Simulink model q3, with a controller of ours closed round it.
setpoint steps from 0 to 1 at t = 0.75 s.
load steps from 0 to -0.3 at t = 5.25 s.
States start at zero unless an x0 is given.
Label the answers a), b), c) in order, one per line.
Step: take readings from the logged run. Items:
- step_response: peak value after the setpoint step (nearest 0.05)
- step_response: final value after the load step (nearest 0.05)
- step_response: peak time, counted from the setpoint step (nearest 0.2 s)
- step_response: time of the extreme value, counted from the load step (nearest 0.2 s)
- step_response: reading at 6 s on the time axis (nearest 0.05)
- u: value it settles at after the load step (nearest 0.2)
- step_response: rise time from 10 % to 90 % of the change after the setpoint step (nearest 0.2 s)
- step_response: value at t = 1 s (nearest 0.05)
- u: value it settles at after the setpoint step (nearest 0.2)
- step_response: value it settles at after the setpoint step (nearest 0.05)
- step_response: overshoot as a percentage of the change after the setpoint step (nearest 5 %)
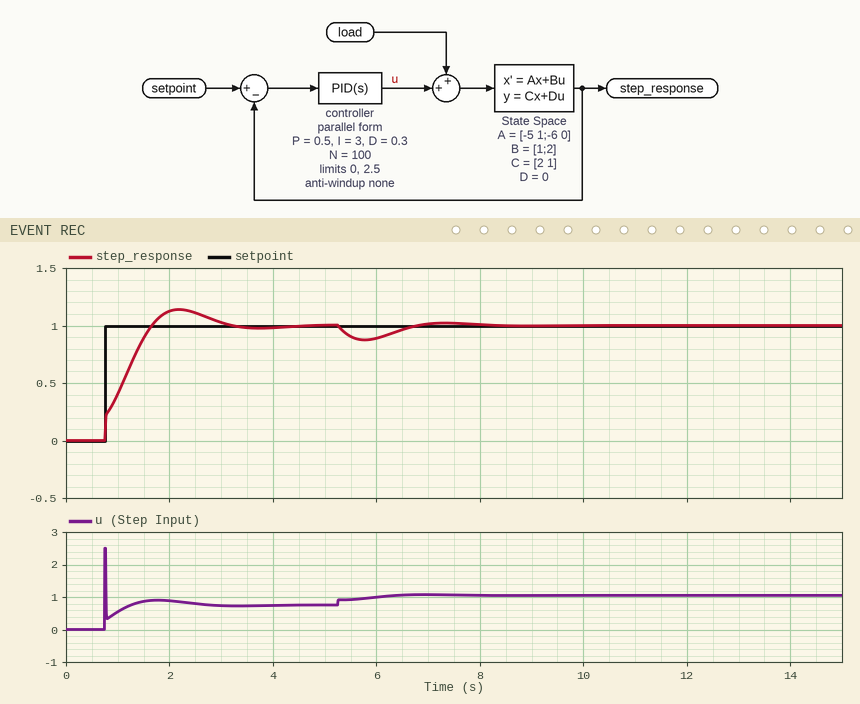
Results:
a) 1.15
b) 1.00
c) 1.4 s
d) 0.6 s
e) 0.90
f) 1.0
g) 0.8 s
h) 0.40
i) 0.8
j) 1.00
k) 15 %
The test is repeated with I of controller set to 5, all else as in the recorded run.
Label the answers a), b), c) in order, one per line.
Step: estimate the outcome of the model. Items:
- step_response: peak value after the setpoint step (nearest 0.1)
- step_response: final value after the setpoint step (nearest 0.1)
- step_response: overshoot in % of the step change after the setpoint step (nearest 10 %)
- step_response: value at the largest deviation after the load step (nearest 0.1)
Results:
a) 1.2
b) 1.0
c) 20 %
d) 0.9
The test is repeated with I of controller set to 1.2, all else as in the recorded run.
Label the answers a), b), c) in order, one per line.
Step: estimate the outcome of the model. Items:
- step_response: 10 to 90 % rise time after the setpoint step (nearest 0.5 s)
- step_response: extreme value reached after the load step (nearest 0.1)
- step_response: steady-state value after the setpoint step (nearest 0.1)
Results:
a) 1.5 s
b) 0.8
c) 1.0
